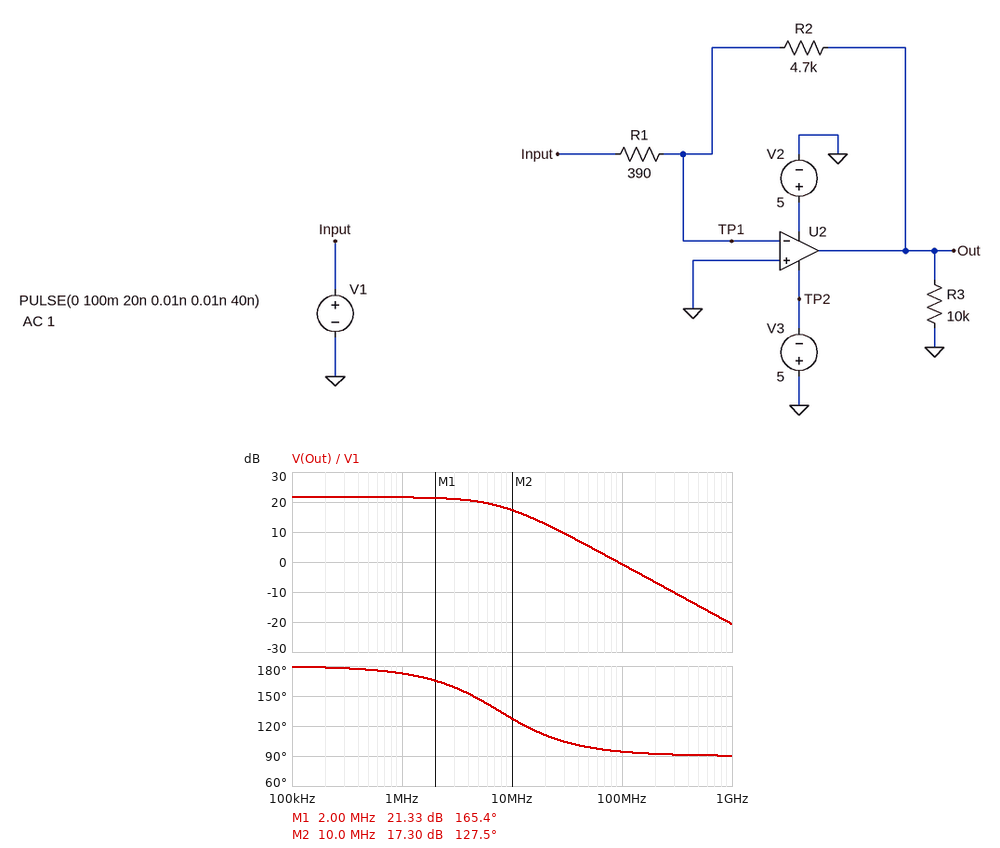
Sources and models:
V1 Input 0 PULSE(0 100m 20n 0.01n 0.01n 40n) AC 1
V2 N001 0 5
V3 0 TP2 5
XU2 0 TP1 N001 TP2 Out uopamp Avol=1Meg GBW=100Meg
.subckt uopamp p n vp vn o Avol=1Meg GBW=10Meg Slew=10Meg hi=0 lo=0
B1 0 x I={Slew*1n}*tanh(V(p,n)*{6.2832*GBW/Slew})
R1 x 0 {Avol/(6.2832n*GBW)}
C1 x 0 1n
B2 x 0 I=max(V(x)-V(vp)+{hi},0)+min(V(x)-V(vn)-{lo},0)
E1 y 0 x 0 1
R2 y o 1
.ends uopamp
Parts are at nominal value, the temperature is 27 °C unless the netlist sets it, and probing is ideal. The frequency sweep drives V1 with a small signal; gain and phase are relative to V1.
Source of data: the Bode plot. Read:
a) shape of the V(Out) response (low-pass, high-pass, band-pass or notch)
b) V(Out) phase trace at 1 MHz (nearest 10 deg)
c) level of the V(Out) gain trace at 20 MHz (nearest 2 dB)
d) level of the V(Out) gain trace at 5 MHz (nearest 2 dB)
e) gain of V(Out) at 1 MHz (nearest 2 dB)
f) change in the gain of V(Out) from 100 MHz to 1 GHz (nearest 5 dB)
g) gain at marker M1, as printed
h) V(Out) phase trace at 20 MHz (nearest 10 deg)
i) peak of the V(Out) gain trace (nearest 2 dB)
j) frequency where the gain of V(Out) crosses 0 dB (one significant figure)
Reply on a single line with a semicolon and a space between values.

low-pass; 170 deg; 12 dB; 20 dB; 22 dB; -20 dB; 21.33 dB; 110 deg; 22 dB; 90 MHz
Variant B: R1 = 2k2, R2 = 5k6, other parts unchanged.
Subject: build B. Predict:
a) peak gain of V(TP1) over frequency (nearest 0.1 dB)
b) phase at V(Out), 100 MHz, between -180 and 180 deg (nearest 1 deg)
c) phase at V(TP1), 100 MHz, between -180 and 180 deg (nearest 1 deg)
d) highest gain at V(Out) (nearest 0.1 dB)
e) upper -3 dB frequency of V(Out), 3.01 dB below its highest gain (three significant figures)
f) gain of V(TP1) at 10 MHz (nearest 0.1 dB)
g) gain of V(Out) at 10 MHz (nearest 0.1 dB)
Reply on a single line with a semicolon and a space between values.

-2.9 dB; 106 deg; 16 deg; 8.1 dB; 28.2 MHz; -12.4 dB; 7.6 dB
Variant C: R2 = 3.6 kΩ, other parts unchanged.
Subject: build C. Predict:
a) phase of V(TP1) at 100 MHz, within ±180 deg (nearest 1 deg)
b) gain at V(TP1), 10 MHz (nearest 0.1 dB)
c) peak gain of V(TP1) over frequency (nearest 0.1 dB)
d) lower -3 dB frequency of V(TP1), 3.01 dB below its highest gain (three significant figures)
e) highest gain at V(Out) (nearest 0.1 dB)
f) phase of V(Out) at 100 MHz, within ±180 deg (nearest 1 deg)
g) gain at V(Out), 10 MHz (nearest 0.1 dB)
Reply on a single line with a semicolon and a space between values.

6 deg; -3.8 dB; -0.9 dB; 9.77 MHz; 19.3 dB; 96 deg; 16.2 dB
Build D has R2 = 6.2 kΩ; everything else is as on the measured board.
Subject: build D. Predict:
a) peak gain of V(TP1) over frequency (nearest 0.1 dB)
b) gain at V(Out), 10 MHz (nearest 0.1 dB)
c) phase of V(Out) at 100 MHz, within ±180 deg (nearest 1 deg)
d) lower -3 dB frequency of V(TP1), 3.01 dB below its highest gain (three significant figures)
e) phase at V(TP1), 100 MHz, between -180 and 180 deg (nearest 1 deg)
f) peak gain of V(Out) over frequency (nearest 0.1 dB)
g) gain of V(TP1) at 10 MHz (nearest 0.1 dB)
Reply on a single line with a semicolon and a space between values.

-0.5 dB; 18.2 dB; 93 deg; 5.92 MHz; 3 deg; 24.0 dB; -1.8 dB
